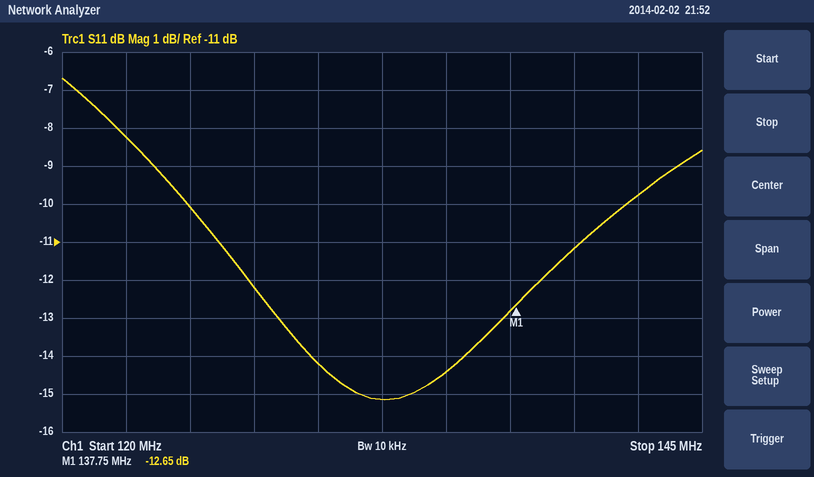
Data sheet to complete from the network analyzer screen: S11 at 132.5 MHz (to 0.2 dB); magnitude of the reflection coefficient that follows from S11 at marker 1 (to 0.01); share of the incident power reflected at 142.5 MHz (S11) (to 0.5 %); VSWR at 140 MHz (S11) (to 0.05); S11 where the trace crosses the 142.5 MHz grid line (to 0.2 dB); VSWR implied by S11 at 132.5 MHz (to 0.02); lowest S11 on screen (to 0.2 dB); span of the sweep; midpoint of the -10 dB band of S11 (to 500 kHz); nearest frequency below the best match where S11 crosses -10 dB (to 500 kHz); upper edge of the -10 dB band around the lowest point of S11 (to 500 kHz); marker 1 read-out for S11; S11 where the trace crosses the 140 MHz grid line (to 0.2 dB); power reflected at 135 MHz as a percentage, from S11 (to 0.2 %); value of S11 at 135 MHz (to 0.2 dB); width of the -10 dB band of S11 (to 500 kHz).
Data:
-15.2 dB
0.23
10.5 %
1.75
-9.8 dB
1.42
-15.2 dB
25 MHz
133.5 MHz
125.0 MHz
142.0 MHz
-12.65 dB
-11.2 dB
3.6 %
-14.4 dB
17.0 MHz
